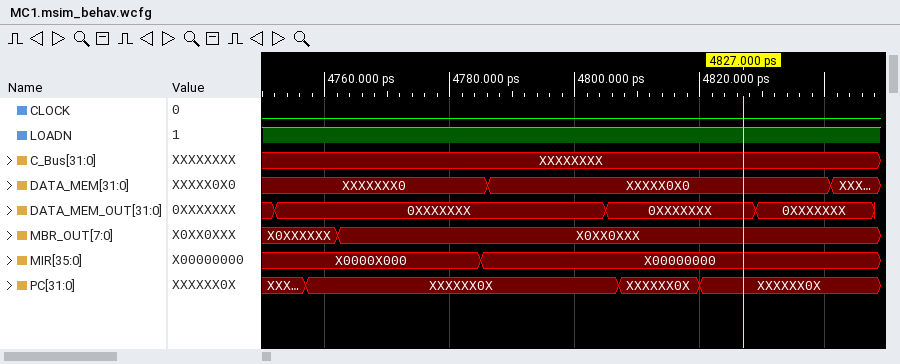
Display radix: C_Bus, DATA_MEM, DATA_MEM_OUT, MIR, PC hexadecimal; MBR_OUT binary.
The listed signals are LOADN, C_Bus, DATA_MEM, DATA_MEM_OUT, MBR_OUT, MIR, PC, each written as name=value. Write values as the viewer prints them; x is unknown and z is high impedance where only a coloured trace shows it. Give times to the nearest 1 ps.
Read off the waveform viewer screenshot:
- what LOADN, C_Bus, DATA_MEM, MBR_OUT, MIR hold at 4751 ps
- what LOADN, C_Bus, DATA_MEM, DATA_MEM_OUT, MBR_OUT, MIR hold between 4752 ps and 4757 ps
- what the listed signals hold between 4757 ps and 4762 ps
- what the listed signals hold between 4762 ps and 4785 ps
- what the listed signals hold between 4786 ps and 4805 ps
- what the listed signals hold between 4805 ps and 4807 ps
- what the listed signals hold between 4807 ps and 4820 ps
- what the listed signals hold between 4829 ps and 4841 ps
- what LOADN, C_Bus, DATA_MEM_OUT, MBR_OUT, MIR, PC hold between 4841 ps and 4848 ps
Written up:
LOADN=1, C_Bus=XXXXXXXX, DATA_MEM=XXXXXXX0, MBR_OUT=X0XXXXXX, MIR=X0000X000
LOADN=1, C_Bus=XXXXXXXX, DATA_MEM=XXXXXXX0, DATA_MEM_OUT=0XXXXXXX, MBR_OUT=X0XXXXXX, MIR=X0000X000
LOADN=1, C_Bus=XXXXXXXX, DATA_MEM=XXXXXXX0, DATA_MEM_OUT=0XXXXXXX, MBR_OUT=X0XXXXXX, MIR=X0000X000, PC=XXXXXX0X
LOADN=1, C_Bus=XXXXXXXX, DATA_MEM=XXXXXXX0, DATA_MEM_OUT=0XXXXXXX, MBR_OUT=X0XX0XXX, MIR=X0000X000, PC=XXXXXX0X
LOADN=1, C_Bus=XXXXXXXX, DATA_MEM=XXXXX0X0, DATA_MEM_OUT=0XXXXXXX, MBR_OUT=X0XX0XXX, MIR=X00000000, PC=XXXXXX0X
LOADN=1, C_Bus=XXXXXXXX, DATA_MEM=XXXXX0X0, DATA_MEM_OUT=0XXXXXXX, MBR_OUT=X0XX0XXX, MIR=X00000000, PC=XXXXXX0X
LOADN=1, C_Bus=XXXXXXXX, DATA_MEM=XXXXX0X0, DATA_MEM_OUT=0XXXXXXX, MBR_OUT=X0XX0XXX, MIR=X00000000, PC=XXXXXX0X
LOADN=1, C_Bus=XXXXXXXX, DATA_MEM=XXXXX0X0, DATA_MEM_OUT=0XXXXXXX, MBR_OUT=X0XX0XXX, MIR=X00000000, PC=XXXXXX0X
LOADN=1, C_Bus=XXXXXXXX, DATA_MEM_OUT=0XXXXXXX, MBR_OUT=X0XX0XXX, MIR=X00000000, PC=XXXXXX0X
